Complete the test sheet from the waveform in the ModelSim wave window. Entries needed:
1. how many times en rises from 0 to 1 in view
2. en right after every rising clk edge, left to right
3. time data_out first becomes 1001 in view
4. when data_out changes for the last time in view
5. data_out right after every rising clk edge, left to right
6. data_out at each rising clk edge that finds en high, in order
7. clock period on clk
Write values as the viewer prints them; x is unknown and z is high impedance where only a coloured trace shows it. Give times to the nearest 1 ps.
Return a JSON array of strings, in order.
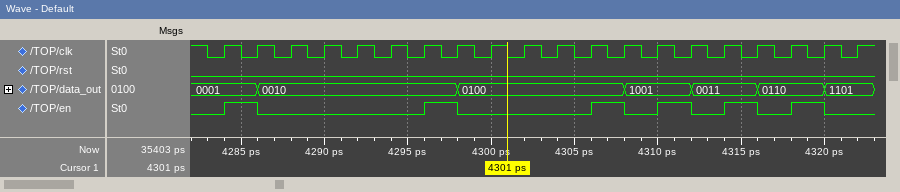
["6", "1 0 0 0 0 0 1 0 0 0 0 1 0 1 0 1 0 1 0 0", "4308 ps", "4320 ps", "0001, 0010, 0010, 0010, 0010, 0010, 0010, 0100, 0100, 0100, 0100, 0100, 1001, 1001, 0011, 0011, 0110, 0110, 1101, 1101", "0001, 0010, 0100, 1001, 0011, 0110", "2 ps"]
